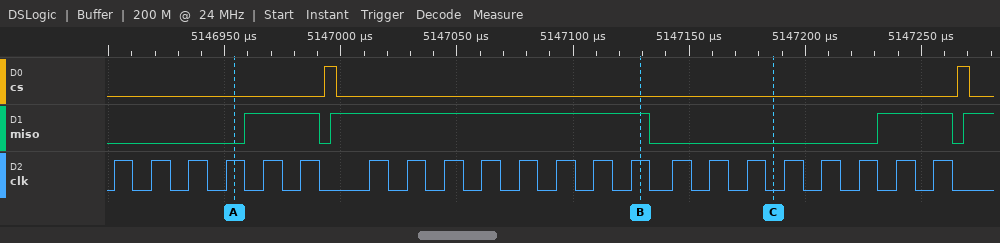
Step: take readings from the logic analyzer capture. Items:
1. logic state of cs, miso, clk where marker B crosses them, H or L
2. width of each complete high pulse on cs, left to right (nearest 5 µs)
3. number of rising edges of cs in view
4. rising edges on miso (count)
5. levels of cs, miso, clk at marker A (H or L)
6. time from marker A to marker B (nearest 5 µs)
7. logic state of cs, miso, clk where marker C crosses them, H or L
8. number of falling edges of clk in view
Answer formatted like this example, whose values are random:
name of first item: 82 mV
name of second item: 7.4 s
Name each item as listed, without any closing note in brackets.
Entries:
logic state of cs, miso, clk where marker B crosses them, H or L: cs=L, miso=H, clk=H
width of each complete high pulse on cs, left to right: 5 µs, 5 µs
number of rising edges of cs in view: 2
rising edges on miso: 4
levels of cs, miso, clk at marker A: cs=L, miso=L, clk=H
time from marker A to marker B: 175 µs
logic state of cs, miso, clk where marker C crosses them, H or L: cs=L, miso=L, clk=L
number of falling edges of clk in view: 22
